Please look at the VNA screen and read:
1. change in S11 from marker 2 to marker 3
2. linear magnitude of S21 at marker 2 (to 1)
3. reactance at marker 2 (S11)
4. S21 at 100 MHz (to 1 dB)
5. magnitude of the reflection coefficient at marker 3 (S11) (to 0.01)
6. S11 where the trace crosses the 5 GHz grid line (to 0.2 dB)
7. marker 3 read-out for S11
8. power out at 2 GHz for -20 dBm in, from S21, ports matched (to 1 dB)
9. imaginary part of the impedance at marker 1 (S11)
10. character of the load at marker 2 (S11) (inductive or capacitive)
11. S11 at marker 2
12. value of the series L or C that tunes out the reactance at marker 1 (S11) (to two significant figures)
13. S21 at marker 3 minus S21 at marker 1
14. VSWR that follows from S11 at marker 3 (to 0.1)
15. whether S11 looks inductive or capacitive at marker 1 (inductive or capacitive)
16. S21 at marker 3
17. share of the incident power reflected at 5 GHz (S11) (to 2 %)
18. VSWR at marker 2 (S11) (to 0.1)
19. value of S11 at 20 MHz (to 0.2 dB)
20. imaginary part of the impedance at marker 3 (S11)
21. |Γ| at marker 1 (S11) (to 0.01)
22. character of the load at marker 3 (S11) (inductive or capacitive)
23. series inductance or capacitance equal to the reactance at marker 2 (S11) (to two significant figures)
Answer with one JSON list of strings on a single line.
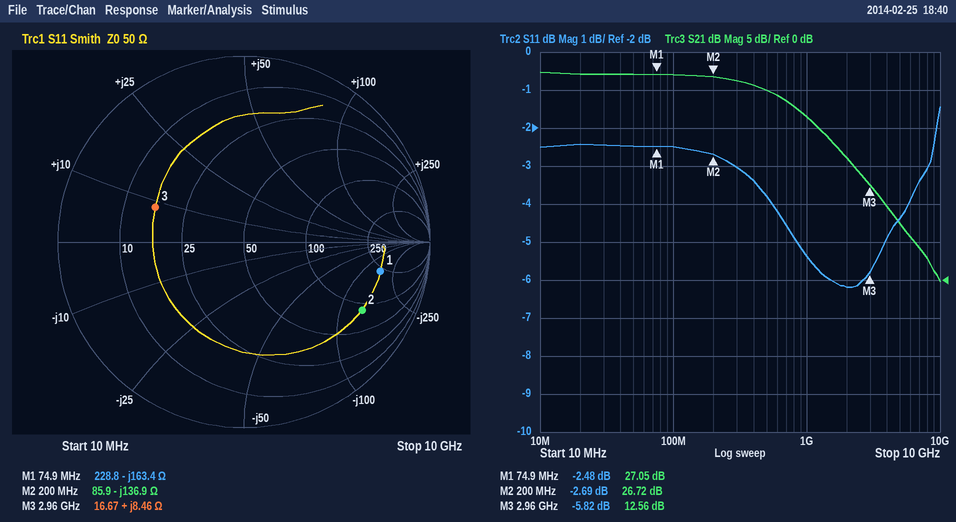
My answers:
["-3.13 dB", "22", "-136.9 Ω", "27 dB", "0.51", "-4.4 dB", "-5.82 dB", "-4 dBm", "-163.4 Ω", "capacitive", "-2.69 dB", "350 nH", "-14.49 dB", "3.1", "capacitive", "12.56 dB", "36 %", "6.5", "-2.4 dB", "+8.46 Ω", "0.75", "inductive", "5.8 pF"]
